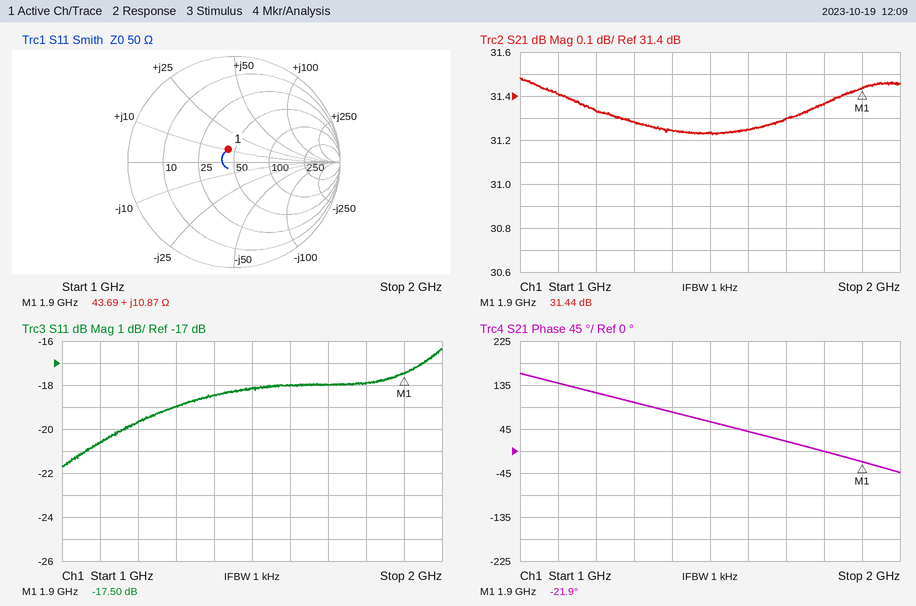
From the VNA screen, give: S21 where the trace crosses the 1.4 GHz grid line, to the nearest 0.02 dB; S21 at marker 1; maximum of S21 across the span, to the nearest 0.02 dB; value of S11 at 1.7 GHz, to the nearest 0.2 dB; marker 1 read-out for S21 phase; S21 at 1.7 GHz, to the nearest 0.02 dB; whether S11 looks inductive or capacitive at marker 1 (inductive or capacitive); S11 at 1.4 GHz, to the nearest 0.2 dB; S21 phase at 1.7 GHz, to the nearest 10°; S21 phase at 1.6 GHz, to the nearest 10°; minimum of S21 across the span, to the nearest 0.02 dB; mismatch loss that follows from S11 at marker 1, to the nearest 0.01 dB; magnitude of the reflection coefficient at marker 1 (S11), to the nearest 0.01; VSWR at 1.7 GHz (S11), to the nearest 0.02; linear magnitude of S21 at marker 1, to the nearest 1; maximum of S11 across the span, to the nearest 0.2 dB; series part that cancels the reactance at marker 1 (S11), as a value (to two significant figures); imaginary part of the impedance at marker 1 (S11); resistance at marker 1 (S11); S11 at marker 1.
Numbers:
31.24 dB
31.44 dB
31.48 dB
-18.0 dB
-21.9°
31.30 dB
inductive
-18.4 dB
20°
40°
31.22 dB
0.08 dB
0.13
1.28
37
-16.4 dB
7.7 pF
+10.87 Ω
43.69 Ω
-17.50 dB
